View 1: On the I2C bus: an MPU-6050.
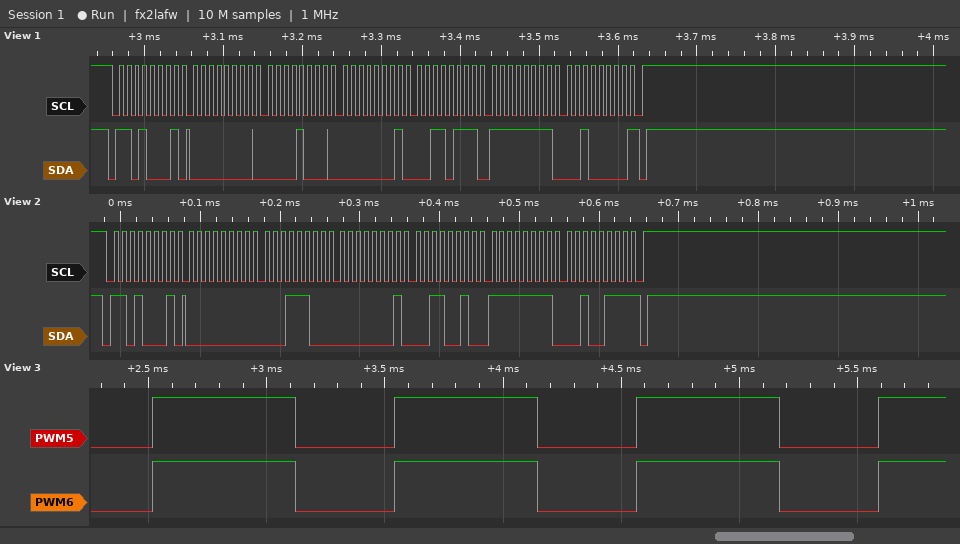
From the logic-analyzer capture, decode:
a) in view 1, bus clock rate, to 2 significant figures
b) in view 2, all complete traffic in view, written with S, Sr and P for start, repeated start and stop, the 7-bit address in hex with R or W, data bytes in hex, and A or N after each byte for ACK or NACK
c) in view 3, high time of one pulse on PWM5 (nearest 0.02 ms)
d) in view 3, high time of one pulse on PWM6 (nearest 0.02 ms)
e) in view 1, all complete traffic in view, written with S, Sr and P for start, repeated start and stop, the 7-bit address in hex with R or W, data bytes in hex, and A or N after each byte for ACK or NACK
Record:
100 kHz
S 68R A 00 A 1C A 01 A 32 A FF A 27 N P
0.60 ms
0.60 ms
S 68R A 00 A 08 A 01 A 37 A FF A 20 N P
